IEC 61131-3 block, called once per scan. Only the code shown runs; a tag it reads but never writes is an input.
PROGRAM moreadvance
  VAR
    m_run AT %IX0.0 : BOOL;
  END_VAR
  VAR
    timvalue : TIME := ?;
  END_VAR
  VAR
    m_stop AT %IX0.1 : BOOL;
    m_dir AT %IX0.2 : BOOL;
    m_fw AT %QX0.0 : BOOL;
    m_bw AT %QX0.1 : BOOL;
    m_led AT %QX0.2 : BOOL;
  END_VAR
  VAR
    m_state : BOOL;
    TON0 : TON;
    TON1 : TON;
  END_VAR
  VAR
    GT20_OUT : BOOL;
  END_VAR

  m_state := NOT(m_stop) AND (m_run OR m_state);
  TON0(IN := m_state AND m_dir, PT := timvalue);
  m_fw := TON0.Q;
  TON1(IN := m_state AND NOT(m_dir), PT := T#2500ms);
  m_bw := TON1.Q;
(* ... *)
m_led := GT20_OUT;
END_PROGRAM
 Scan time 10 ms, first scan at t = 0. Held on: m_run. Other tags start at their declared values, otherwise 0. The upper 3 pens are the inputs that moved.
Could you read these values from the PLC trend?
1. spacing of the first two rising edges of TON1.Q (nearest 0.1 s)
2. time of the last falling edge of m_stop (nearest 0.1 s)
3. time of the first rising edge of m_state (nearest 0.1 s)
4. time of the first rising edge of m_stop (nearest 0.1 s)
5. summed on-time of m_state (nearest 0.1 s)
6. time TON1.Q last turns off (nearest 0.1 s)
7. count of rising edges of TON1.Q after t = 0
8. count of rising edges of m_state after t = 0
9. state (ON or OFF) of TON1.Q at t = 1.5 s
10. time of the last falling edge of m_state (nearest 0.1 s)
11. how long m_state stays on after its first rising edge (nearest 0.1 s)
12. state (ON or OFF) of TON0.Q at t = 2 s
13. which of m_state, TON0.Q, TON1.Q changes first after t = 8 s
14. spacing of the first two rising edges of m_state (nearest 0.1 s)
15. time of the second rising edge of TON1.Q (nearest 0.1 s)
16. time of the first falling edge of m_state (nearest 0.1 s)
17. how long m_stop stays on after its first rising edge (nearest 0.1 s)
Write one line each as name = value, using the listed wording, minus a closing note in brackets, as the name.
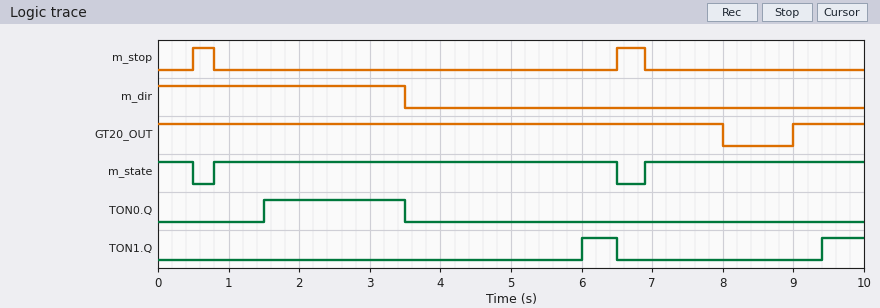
spacing of the first two rising edges of TON1.Q = 3.4 s
time of the last falling edge of m_stop = 6.9 s
time of the first rising edge of m_state = 0.8 s
time of the first rising edge of m_stop = 0.5 s
summed on-time of m_state = 9.3 s
time TON1.Q last turns off = 6.5 s
count of rising edges of TON1.Q after t = 0 = 2
count of rising edges of m_state after t = 0 = 2
state (ON or OFF) of TON1.Q at t = 1.5 s = OFF
time of the last falling edge of m_state = 6.5 s
how long m_state stays on after its first rising edge = 5.7 s
state (ON or OFF) of TON0.Q at t = 2 s = ON
which of m_state, TON0.Q, TON1.Q changes first after t = 8 s = TON1.Q
spacing of the first two rising edges of m_state = 6.1 s
time of the second rising edge of TON1.Q = 9.4 s
time of the first falling edge of m_state = 0.5 s
how long m_stop stays on after its first rising edge = 0.3 s
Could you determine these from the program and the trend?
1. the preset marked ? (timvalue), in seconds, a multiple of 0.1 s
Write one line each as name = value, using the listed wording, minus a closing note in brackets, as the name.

the preset marked ? (timvalue), in seconds, a multiple of 0.1 s = 0.7 s
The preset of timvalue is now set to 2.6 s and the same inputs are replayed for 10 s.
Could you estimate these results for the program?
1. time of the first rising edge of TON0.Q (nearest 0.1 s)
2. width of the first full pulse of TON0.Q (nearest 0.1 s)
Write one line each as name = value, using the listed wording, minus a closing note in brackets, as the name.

time of the first rising edge of TON0.Q = 3.4 s
width of the first full pulse of TON0.Q = 0.1 s
